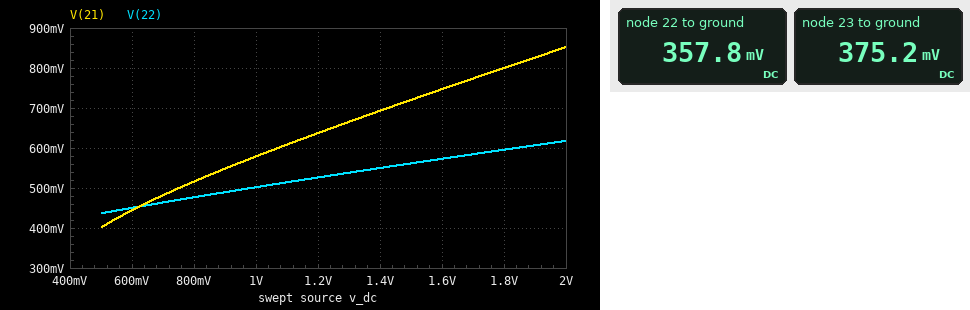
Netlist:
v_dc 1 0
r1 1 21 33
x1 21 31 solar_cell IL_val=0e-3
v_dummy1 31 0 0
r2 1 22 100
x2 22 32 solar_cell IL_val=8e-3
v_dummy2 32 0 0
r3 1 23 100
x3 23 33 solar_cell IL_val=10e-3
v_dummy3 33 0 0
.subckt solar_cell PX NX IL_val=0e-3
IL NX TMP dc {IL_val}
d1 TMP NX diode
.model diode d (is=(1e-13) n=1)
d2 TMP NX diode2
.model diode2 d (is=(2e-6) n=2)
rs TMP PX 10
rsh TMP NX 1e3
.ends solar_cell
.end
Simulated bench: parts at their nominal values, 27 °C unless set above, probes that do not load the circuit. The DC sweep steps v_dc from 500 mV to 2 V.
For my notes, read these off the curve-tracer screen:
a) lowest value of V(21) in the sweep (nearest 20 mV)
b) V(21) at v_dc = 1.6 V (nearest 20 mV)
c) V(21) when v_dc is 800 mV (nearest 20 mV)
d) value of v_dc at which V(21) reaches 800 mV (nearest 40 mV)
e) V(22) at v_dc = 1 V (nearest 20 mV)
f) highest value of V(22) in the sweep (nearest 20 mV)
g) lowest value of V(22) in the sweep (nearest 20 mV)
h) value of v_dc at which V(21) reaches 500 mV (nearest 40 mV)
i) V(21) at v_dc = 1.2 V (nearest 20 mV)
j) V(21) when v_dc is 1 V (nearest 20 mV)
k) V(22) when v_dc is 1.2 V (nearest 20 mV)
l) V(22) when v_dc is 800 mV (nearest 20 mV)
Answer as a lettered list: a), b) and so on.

a) 400 mV
b) 740 mV
c) 520 mV
d) 1.80 V
e) 500 mV
f) 620 mV
g) 440 mV
h) 760 mV
i) 640 mV
j) 580 mV
k) 520 mV
l) 480 mV
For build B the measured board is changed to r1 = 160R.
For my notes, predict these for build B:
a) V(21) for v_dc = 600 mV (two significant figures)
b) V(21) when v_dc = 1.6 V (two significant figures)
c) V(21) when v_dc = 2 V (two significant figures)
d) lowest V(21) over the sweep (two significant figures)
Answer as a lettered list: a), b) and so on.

a) 350 mV
b) 490 mV
c) 530 mV
d) 320 mV
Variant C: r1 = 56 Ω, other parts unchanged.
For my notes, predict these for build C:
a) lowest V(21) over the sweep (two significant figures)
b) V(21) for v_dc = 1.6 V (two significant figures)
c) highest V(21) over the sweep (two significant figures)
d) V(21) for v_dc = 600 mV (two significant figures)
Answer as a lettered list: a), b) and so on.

a) 380 mV
b) 640 mV
c) 710 mV
d) 410 mV
